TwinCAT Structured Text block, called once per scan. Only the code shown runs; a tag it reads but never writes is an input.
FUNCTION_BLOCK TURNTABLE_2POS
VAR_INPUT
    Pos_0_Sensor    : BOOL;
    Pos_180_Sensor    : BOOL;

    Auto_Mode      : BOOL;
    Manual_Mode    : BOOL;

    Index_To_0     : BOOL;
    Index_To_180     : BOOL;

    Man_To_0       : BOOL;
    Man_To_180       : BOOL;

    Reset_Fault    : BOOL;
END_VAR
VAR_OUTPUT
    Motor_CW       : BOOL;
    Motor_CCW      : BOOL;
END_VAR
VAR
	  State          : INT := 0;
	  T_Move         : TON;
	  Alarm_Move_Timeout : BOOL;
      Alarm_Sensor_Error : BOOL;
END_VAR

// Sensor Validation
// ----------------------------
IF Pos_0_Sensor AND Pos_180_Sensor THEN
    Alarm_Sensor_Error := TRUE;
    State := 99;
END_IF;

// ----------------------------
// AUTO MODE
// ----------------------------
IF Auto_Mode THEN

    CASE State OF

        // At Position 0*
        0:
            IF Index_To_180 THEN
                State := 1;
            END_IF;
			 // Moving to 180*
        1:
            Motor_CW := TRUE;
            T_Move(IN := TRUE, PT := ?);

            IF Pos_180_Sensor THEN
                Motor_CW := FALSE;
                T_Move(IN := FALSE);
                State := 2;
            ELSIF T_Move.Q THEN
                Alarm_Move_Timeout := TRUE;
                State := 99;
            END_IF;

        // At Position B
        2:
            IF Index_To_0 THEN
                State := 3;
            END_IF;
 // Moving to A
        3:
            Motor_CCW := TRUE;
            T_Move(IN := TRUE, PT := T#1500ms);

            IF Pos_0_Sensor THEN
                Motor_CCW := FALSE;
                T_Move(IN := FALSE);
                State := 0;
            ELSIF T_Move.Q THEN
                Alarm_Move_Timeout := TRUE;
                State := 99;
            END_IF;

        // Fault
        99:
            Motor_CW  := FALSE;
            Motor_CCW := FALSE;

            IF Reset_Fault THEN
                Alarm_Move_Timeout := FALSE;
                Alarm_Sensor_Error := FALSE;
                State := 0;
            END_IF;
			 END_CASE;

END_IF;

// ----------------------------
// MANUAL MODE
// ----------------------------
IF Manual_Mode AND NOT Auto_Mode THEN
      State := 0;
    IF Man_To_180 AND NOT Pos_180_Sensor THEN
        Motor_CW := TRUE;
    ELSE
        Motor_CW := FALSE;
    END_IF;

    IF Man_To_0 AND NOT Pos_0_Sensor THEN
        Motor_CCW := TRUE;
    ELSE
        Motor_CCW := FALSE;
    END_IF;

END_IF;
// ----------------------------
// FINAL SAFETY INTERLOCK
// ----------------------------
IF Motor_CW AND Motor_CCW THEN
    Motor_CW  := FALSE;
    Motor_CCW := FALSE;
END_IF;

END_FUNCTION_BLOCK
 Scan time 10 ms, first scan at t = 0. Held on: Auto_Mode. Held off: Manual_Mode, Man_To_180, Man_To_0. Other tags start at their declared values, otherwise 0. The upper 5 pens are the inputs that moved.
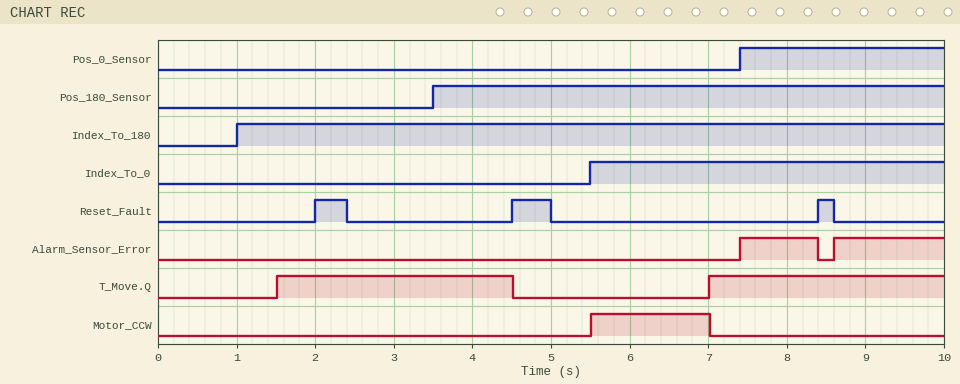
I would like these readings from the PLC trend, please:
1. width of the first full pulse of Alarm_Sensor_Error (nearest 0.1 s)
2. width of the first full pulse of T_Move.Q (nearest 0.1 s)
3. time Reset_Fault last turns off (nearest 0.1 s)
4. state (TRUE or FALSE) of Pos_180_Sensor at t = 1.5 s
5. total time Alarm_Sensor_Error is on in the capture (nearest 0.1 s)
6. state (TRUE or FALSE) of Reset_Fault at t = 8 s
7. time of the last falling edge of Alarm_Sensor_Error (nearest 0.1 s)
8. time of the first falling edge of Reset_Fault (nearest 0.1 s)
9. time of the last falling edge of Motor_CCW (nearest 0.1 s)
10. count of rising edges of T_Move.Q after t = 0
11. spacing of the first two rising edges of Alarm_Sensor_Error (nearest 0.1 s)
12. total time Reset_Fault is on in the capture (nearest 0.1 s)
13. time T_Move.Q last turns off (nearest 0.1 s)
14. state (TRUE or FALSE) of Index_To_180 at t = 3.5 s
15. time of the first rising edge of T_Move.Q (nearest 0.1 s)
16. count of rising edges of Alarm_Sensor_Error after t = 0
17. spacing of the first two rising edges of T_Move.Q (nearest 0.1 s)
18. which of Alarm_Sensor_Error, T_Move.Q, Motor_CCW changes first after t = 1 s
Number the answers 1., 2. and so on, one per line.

1. 1.0 s
2. 3.0 s
3. 8.6 s
4. FALSE
5. 2.4 s
6. FALSE
7. 8.4 s
8. 2.4 s
9. 7.0 s
10. 2
11. 1.2 s
12. 1.1 s
13. 4.5 s
14. TRUE
15. 1.5 s
16. 2
17. 5.5 s
18. T_Move.Q
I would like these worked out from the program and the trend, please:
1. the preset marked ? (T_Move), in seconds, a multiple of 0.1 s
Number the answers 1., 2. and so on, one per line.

1. 0.5 s
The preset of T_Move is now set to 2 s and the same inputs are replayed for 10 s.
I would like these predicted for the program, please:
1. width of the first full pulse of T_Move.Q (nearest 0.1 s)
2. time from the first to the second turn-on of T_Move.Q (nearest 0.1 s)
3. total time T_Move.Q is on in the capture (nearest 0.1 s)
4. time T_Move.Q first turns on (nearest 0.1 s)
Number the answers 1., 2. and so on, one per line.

1. 1.5 s
2. 4.0 s
3. 4.5 s
4. 3.0 s
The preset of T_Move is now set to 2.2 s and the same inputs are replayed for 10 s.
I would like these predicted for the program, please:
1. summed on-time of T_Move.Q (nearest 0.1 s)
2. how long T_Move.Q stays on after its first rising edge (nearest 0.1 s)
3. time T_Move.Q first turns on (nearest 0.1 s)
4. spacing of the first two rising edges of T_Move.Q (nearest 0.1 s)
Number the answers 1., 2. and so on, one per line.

1. 4.3 s
2. 1.3 s
3. 3.2 s
4. 3.8 s
